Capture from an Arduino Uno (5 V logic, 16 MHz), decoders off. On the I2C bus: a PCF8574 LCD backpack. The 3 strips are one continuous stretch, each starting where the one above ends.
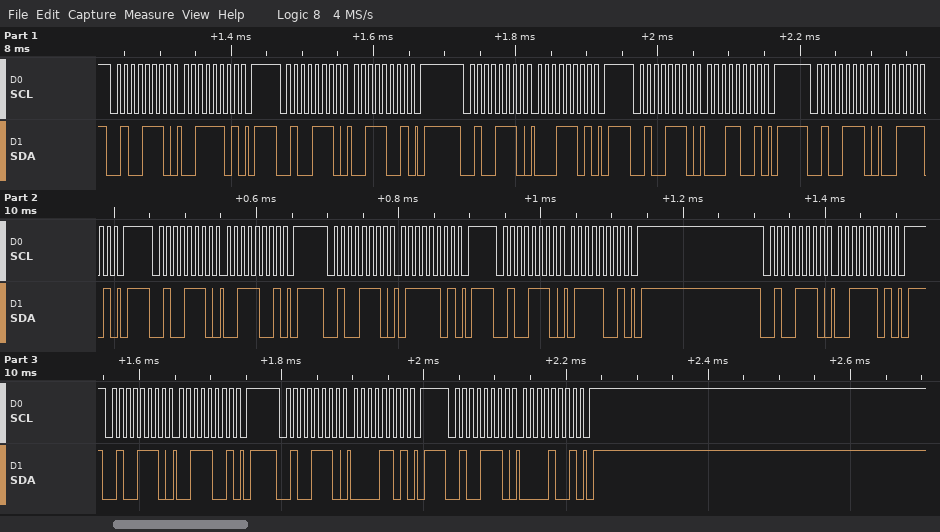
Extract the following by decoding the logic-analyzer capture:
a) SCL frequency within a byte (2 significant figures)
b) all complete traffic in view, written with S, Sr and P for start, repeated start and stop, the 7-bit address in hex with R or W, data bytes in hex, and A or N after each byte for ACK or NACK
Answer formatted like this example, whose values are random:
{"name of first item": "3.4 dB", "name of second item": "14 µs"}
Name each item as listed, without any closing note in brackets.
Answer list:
{"SCL frequency within a byte": "100 kHz", "all complete traffic in view, written with S, Sr and P for start, repeated start and stop, the 7-bit address in hex with R or W, data bytes in hex, and A or N after each byte for ACK or NACK": "S 27W A 3D A P S 27W A 39 A P S 27W A 1D A P S 27W A 19 A P S 27W A 3D A P S 27W A 39 A P S 27W A 7D A P S 27W A 79 A P S 27W A 3D A P S 27W A 39 A P S 27W A 0D A P S 27W A 09 A P"}
